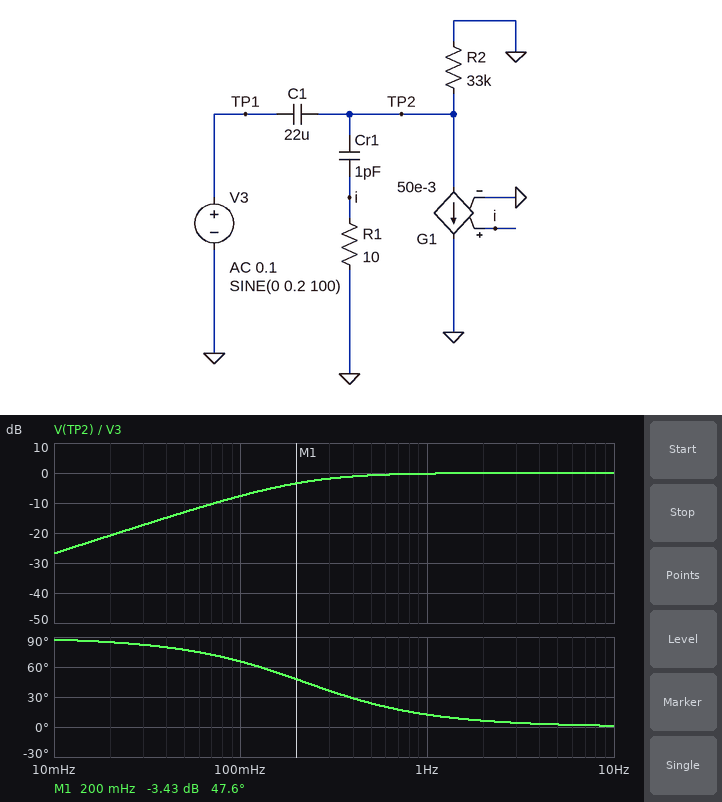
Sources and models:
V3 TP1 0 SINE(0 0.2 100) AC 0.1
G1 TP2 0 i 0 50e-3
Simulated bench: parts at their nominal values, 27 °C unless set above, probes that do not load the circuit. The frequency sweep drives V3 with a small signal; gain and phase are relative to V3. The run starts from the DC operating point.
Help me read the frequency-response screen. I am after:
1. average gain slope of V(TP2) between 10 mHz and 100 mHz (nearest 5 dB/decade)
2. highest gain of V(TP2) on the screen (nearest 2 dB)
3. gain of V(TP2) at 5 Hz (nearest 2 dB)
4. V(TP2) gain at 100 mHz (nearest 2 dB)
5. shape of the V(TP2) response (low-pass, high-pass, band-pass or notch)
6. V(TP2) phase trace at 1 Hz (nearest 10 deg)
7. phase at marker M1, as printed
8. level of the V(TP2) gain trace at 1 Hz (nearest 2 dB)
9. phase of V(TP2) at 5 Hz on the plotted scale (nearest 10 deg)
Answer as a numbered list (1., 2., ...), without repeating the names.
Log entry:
1. 20 dB/decade
2. 0 dB
3. 0 dB
4. -8 dB
5. high-pass
6. 10 deg
7. 47.6 deg
8. 0 dB
9. 0 deg
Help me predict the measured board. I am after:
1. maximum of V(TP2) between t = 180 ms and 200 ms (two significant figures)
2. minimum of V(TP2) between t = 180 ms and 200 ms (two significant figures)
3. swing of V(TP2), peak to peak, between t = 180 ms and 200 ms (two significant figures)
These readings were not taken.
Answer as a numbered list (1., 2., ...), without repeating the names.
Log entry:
1. 200 mV
2. -200 mV
3. 400 mV
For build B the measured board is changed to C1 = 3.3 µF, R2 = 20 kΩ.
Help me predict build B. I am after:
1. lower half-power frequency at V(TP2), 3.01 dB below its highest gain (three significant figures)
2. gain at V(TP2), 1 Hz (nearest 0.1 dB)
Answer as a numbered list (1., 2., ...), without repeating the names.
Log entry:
1. 2.41 Hz
2. -8.3 dB
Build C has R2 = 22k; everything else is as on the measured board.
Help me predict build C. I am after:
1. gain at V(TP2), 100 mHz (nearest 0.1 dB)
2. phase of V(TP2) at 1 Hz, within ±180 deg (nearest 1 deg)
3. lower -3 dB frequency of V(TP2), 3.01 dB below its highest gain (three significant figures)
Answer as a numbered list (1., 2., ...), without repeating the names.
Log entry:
1. -10.7 dB
2. 18 deg
3. 329 mHz
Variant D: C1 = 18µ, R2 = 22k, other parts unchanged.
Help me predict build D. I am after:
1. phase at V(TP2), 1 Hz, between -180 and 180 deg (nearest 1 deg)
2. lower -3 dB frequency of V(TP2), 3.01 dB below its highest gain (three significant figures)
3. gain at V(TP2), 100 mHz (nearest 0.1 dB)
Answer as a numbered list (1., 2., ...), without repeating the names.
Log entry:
1. 22 deg
2. 402 mHz
3. -12.3 dB
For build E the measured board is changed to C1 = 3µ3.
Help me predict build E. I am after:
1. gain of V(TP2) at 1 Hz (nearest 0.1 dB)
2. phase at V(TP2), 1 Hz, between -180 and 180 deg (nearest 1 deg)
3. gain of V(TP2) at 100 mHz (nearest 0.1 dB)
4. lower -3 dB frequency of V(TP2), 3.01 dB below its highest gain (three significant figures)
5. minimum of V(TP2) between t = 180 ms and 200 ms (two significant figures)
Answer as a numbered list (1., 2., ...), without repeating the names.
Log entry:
1. -5.0 dB
2. 56 deg
3. -23.3 dB
4. 1.46 Hz
5. -200 mV
